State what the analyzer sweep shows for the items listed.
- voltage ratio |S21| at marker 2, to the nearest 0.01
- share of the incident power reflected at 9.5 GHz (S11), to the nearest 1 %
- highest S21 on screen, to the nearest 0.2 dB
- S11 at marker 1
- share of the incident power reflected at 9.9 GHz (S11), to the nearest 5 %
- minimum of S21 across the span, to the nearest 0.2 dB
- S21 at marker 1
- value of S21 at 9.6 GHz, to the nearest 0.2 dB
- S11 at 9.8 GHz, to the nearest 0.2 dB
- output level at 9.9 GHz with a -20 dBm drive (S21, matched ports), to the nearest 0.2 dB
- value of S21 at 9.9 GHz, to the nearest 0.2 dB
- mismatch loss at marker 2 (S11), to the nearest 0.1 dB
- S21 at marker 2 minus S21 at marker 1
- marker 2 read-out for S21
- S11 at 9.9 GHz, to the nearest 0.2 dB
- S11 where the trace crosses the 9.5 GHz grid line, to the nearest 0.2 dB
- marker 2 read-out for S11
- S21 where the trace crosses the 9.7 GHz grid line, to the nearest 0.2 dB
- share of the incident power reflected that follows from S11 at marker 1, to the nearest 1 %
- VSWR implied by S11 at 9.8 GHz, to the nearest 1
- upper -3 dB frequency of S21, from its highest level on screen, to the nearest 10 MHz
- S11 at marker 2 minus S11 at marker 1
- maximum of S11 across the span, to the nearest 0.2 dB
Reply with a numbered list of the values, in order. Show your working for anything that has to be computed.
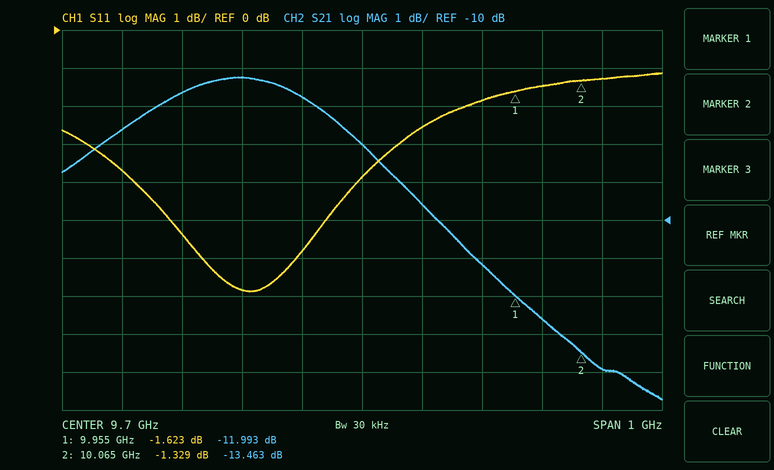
1. 10^(-13.463/20) ≈ 0.21
2. 10^(-6.8/10) ≈ 21 %
3. -6.2 dB
4. -1.623 dB
5. 10^(-1.8/10) ≈ 66.1 %, so 65 % to the nearest 5 %
6. -14.8 dB
7. -11.993 dB
8. -6.8 dB
9. -2.6 dB
10. -20 dBm + (-11.2 dB) = -31.2 dBm
11. -11.2 dB
12. −10 log10(1 − 10^(-1.329/10)) ≈ 5.8 dB
13. -13.463 − (-11.993) = -1.470 dB
14. -13.463 dB
15. -1.8 dB
16. -6.8 dB
17. -1.329 dB
18. -8.0 dB
19. 10^(-1.623/10) ≈ 69 %
20. |Γ| = 10^(-2.6/20) = 0.7413; VSWR = (1 + 0.7413)/(1 − 0.7413) ≈ 7
21. 9.78 GHz
22. -1.329 − (-1.623) = 0.294 dB
23. -1.2 dB
